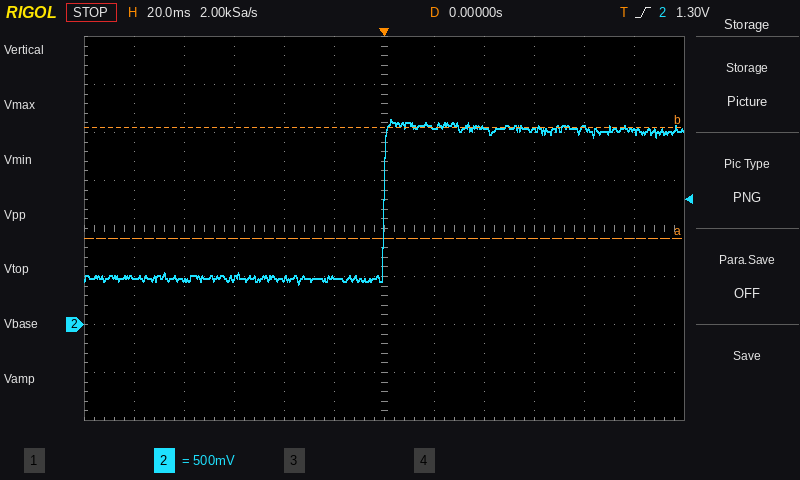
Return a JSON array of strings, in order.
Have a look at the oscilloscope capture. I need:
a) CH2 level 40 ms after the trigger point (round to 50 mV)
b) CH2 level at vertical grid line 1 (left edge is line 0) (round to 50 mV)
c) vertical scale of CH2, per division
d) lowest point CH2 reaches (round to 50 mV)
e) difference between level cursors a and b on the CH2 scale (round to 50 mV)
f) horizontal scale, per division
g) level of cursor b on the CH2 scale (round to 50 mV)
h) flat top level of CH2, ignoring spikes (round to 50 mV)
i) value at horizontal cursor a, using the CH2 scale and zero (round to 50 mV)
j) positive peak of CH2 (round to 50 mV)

["2.05 V", "500 mV", "500 mV", "400 mV", "1.15 V", "20 ms", "2.05 V", "2.05 V", "900 mV", "2.15 V"]
